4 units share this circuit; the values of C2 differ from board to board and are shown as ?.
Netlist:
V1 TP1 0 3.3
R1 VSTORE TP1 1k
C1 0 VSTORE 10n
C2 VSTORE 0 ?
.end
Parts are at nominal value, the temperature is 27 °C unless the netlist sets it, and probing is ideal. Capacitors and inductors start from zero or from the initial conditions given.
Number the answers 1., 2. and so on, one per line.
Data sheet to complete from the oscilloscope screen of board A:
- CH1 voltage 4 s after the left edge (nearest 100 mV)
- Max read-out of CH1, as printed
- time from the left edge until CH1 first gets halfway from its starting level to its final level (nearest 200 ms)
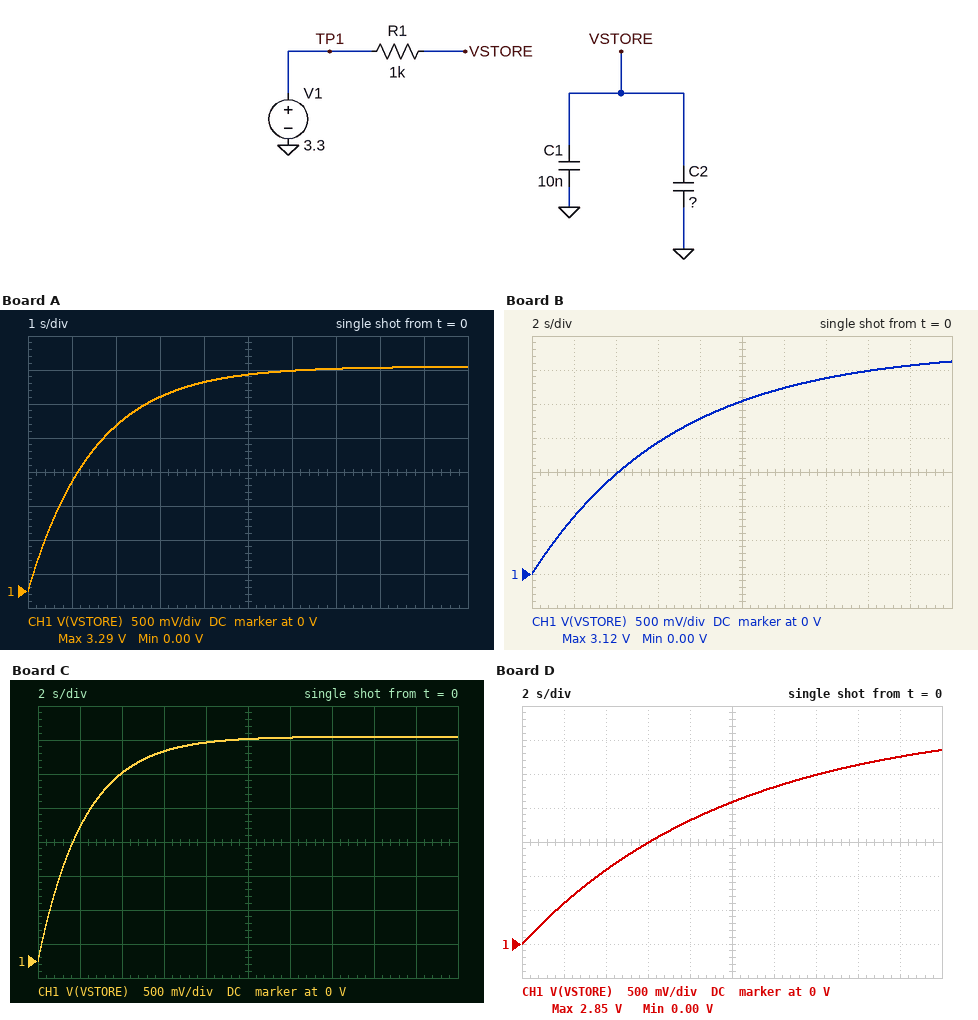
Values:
1. 3.1 V
2. 3.29 V
3. 1.0 s
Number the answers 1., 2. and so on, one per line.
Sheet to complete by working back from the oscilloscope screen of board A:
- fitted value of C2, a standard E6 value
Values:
1. 1.5 mF
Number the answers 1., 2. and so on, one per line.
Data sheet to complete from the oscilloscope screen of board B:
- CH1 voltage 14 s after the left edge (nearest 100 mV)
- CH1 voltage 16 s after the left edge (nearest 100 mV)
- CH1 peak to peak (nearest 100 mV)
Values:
1. 2.9 V
2. 3.0 V
3. 3.1 V
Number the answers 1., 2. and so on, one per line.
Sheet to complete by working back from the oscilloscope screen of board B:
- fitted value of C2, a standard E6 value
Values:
1. 6.8 mF
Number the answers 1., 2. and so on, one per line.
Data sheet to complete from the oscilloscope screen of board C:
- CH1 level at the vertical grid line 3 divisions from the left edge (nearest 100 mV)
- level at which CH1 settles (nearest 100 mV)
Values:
1. 3.1 V
2. 3.3 V
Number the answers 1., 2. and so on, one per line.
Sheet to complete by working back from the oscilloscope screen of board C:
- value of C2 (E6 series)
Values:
1. 2.2 mF
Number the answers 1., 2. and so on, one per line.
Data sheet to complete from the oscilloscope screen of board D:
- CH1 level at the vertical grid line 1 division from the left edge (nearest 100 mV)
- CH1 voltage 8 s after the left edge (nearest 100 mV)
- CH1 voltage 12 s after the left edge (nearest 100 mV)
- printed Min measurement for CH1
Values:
1. 600 mV
2. 1.8 V
3. 2.3 V
4. 0.00 V
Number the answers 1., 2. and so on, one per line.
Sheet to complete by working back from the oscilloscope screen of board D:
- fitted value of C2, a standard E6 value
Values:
1. 10 mF
